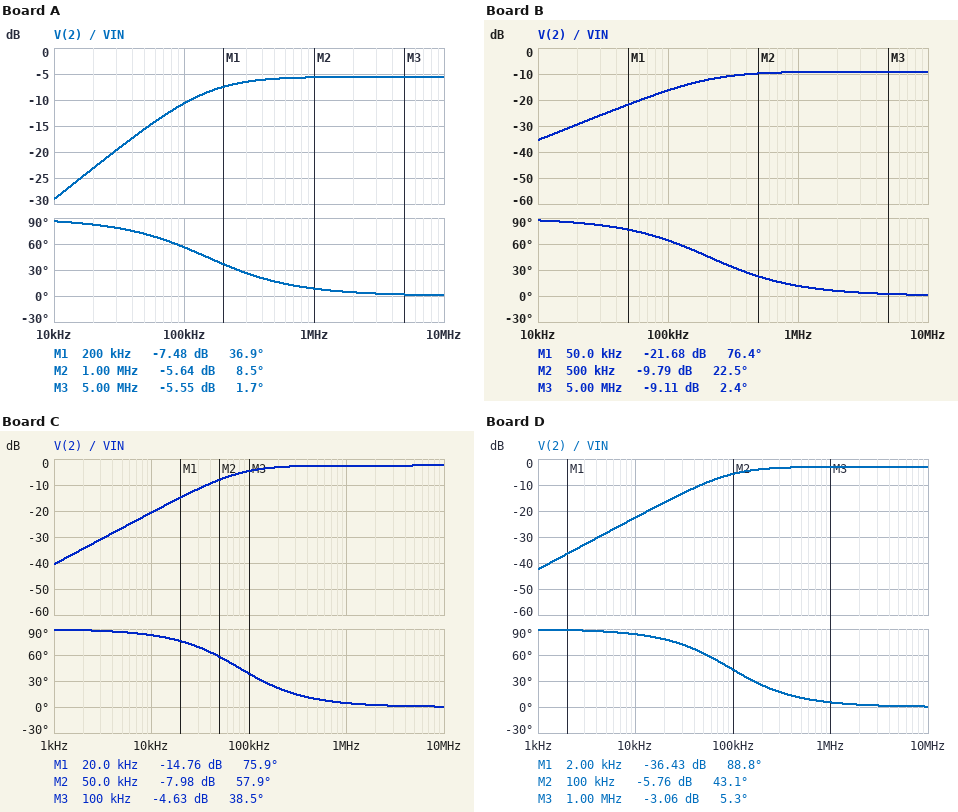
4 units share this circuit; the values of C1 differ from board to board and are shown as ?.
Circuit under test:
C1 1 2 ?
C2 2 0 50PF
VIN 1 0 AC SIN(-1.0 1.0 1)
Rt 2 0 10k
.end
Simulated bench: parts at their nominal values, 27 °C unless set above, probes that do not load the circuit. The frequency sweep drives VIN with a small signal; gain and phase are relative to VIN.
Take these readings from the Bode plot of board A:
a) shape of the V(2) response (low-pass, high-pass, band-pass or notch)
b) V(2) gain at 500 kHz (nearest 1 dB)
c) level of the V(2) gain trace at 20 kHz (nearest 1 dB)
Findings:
high-pass
-6 dB
-23 dB
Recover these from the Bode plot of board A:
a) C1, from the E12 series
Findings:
56 pF
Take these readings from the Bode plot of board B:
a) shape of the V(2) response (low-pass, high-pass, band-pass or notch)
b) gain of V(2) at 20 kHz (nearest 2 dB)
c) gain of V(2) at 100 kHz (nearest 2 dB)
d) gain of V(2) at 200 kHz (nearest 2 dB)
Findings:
high-pass
-30 dB
-16 dB
-12 dB
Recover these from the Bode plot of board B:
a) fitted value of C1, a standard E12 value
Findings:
27 pF
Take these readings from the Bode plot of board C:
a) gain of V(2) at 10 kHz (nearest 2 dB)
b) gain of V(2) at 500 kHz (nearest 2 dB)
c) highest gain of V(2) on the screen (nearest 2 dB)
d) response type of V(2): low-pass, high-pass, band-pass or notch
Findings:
-20 dB
-2 dB
-2 dB
high-pass
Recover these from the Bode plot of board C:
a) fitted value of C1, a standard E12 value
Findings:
150 pF
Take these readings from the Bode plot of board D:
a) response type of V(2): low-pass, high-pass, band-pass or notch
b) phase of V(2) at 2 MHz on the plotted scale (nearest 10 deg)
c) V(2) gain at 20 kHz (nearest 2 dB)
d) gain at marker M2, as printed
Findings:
high-pass
0 deg
-16 dB
-5.76 dB
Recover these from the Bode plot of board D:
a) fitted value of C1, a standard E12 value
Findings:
120 pF
